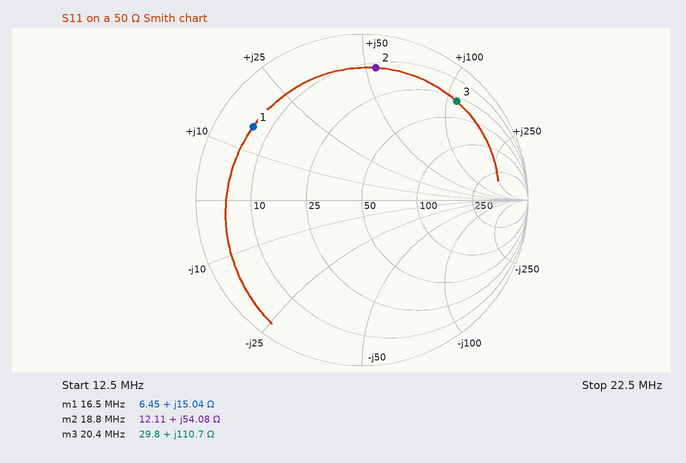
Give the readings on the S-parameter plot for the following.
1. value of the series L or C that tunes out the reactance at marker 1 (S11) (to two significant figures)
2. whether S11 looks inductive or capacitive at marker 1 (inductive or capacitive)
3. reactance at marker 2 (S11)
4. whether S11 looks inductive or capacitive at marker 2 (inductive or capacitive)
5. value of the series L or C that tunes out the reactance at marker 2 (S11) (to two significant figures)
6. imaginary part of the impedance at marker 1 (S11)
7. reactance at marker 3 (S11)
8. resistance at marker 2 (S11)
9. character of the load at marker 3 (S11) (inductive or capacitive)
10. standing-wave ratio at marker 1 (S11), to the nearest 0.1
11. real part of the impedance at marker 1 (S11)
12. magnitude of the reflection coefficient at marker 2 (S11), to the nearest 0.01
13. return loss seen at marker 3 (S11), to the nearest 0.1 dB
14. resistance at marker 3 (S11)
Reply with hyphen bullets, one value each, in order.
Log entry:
- 640 pF
- inductive
- +54.08 Ω
- inductive
- 160 pF
- +15.04 Ω
- +110.7 Ω
- 12.11 Ω
- inductive
- 8.5
- 6.45 Ω
- 0.80
- 1.7 dB
- 29.8 Ω
